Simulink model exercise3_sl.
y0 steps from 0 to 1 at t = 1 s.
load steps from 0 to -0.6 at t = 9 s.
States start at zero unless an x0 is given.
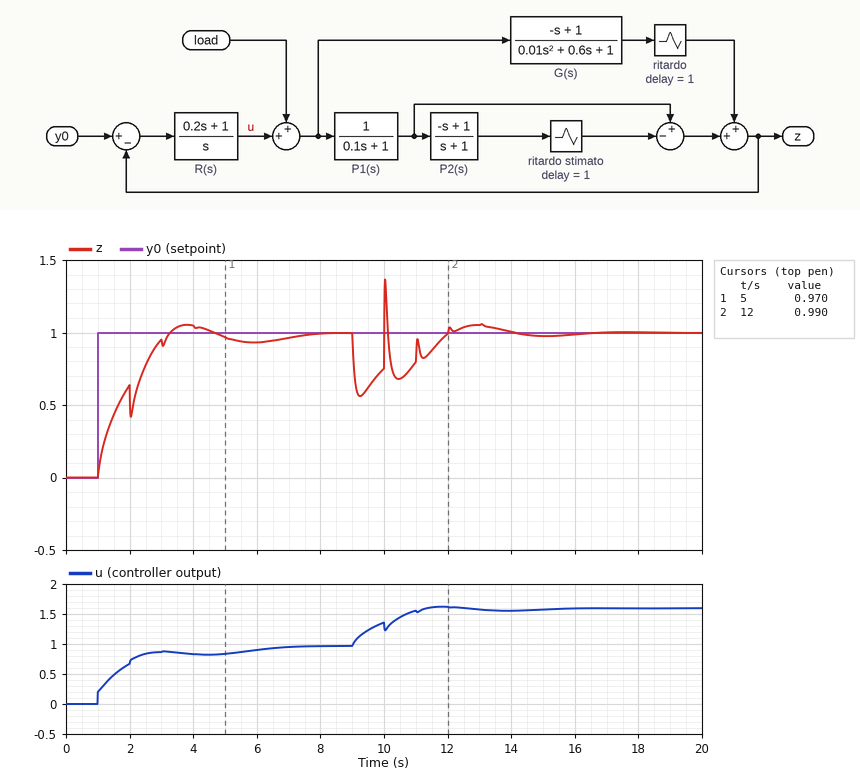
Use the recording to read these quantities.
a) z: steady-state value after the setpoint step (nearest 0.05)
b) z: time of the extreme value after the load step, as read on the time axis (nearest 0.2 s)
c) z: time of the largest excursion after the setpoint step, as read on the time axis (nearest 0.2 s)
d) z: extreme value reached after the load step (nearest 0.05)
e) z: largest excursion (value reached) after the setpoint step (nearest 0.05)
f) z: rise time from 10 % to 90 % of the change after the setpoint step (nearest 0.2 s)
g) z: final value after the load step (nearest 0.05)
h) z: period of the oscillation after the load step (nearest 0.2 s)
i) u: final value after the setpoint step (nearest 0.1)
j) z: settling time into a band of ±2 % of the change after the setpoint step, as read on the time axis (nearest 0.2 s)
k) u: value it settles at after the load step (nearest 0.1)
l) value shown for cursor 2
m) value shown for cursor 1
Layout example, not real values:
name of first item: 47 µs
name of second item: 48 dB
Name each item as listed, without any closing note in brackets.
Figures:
z: steady-state value after the setpoint step: 1.00
z: time of the extreme value after the load step, as read on the time axis: 9.2 s
z: time of the largest excursion after the setpoint step, as read on the time axis: 3.8 s
z: extreme value reached after the load step: 0.55
z: largest excursion (value reached) after the setpoint step: 1.05
z: rise time from 10 % to 90 % of the change after the setpoint step: 1.8 s
z: final value after the load step: 1.00
z: period of the oscillation after the load step: 1.2 s
u: final value after the setpoint step: 1.0
z: settling time into a band of ±2 % of the change after the setpoint step, as read on the time axis: 7.4 s
u: value it settles at after the load step: 1.6
value shown for cursor 2: 0.990
value shown for cursor 1: 0.970
